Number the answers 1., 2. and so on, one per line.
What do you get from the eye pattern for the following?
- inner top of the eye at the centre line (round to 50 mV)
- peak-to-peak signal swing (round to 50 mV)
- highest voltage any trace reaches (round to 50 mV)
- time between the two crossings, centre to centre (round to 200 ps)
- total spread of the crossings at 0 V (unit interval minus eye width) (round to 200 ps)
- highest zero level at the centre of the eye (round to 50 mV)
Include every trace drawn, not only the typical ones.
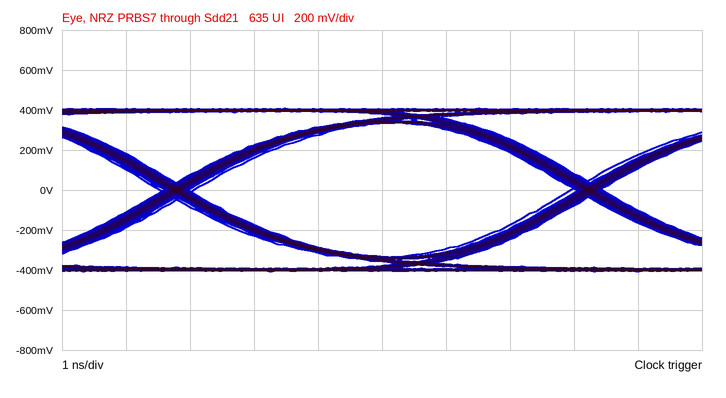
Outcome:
1. 350 mV
2. 800 mV
3. 400 mV
4. 6.4 ns
5. 600 ps
6. -350 mV
